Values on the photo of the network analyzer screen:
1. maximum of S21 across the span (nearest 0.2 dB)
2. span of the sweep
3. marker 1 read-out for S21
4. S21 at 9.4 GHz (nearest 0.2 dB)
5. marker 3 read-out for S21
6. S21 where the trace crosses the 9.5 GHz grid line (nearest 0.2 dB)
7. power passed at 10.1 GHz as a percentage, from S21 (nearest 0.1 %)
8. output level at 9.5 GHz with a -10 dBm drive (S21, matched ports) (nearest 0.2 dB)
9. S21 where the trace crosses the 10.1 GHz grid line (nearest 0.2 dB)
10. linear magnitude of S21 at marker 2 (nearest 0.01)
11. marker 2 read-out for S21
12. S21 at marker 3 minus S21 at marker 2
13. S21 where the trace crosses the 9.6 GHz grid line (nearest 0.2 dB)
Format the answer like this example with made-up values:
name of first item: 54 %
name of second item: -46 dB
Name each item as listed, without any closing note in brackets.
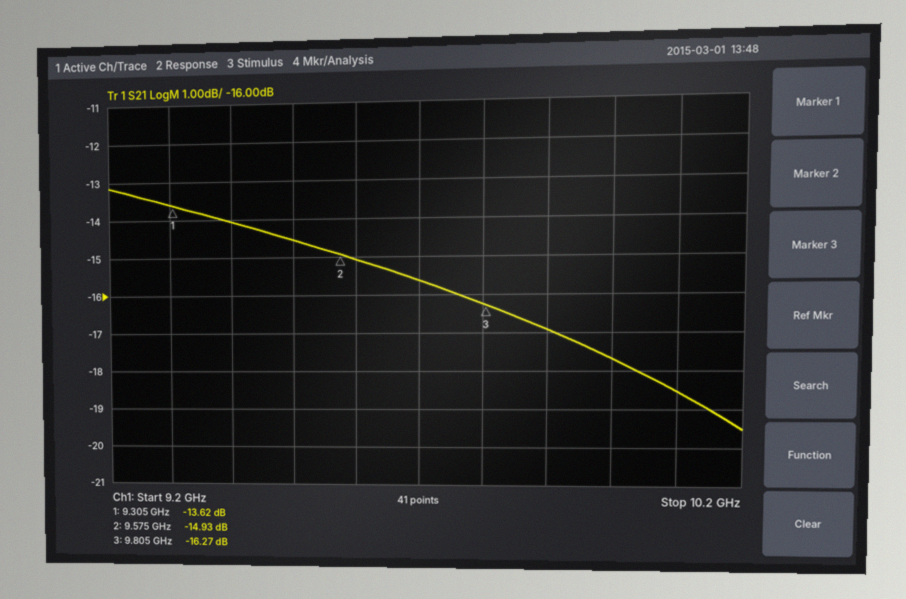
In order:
maximum of S21 across the span: -13.2 dB
span of the sweep: 1 GHz
marker 1 read-out for S21: -13.62 dB
S21 at 9.4 GHz: -14.0 dB
marker 3 read-out for S21: -16.27 dB
S21 where the trace crosses the 9.5 GHz grid line: -14.6 dB
power passed at 10.1 GHz as a percentage, from S21: 1.4 %
output level at 9.5 GHz with a -10 dBm drive (S21, matched ports): -24.6 dBm
S21 where the trace crosses the 10.1 GHz grid line: -18.6 dB
linear magnitude of S21 at marker 2: 0.18
marker 2 read-out for S21: -14.93 dB
S21 at marker 3 minus S21 at marker 2: -1.34 dB
S21 where the trace crosses the 9.6 GHz grid line: -15.0 dB
